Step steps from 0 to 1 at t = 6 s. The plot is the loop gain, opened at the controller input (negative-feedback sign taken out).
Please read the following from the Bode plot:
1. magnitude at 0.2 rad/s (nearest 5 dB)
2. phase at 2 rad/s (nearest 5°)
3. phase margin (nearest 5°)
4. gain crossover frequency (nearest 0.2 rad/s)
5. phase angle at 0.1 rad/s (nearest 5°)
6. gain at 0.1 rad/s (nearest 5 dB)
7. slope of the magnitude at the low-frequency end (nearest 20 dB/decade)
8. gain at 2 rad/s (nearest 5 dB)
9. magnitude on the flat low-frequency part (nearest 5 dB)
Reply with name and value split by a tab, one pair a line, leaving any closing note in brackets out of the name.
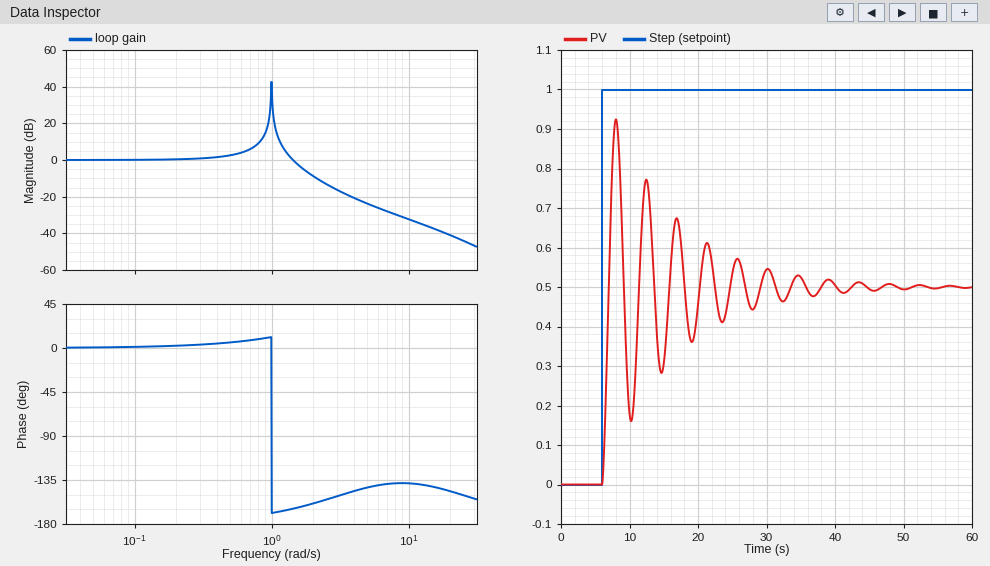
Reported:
magnitude at 0.2 rad/s	0 dB
phase at 2 rad/s	-160°
phase margin	15°
gain crossover frequency	1.4 rad/s
phase angle at 0.1 rad/s	0°
gain at 0.1 rad/s	0 dB
slope of the magnitude at the low-frequency end	0 dB/decade
gain at 2 rad/s	-10 dB
magnitude on the flat low-frequency part	0 dB
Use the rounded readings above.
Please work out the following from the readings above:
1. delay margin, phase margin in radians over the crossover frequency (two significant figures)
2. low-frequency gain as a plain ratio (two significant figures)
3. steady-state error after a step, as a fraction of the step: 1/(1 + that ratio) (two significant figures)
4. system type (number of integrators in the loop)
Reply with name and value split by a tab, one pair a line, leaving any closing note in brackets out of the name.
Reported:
delay margin, phase margin in radians over the crossover frequency	0.19 s
low-frequency gain as a plain ratio	1.0
steady-state error after a step, as a fraction of the step: 1/(1 + that ratio)	0.50
system type	0
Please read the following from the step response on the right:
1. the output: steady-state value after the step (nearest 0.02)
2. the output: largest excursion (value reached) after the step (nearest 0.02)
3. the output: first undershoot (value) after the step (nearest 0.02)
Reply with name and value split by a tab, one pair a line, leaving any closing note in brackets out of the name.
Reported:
the output: steady-state value after the step	0.50
the output: largest excursion (value reached) after the step	0.92
the output: first undershoot (value) after the step	0.16
